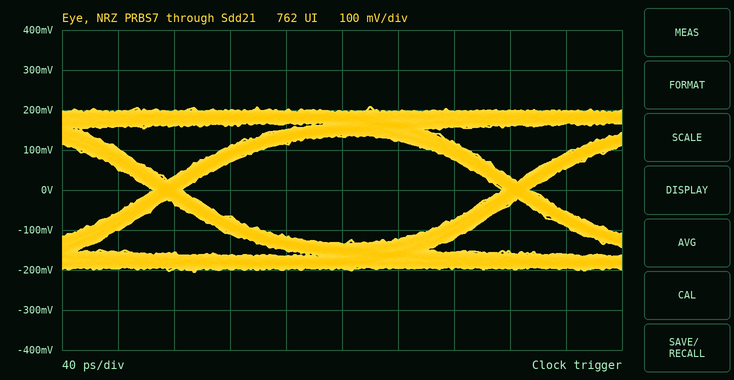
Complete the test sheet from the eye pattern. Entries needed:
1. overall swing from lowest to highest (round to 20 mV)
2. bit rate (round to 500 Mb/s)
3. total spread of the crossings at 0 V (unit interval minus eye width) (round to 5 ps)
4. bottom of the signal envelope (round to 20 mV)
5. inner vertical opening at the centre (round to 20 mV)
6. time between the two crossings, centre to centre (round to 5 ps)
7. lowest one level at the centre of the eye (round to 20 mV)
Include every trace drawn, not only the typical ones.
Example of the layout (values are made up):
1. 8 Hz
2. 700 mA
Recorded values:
1. 420 mV
2. 4.0 Gb/s
3. 20 ps
4. -200 mV
5. 260 mV
6. 250 ps
7. 140 mV
